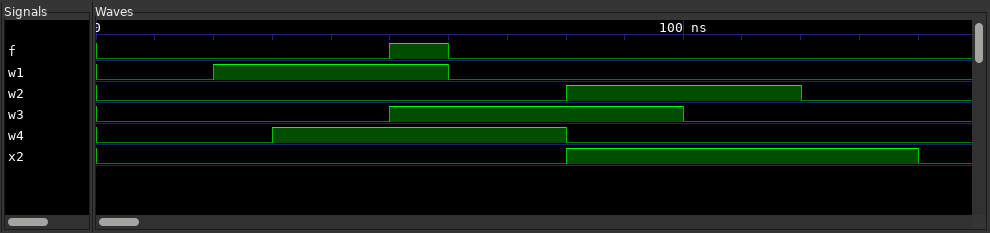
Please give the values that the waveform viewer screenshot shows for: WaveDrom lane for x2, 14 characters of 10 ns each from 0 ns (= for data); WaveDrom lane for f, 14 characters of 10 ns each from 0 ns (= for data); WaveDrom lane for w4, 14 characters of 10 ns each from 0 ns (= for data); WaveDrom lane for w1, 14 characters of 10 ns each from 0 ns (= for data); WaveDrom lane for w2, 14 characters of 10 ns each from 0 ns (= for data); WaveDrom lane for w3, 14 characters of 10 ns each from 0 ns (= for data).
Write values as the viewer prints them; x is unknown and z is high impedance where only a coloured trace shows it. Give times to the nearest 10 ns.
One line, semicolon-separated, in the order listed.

{name: 'x2', wave: '0.......1.....'}; {name: 'f', wave: '0....10.......'}; {name: 'w4', wave: '0..1....0.....'}; {name: 'w1', wave: '0.1...0.......'}; {name: 'w2', wave: '0.......1...0.'}; {name: 'w3', wave: '0....1....0...'}
